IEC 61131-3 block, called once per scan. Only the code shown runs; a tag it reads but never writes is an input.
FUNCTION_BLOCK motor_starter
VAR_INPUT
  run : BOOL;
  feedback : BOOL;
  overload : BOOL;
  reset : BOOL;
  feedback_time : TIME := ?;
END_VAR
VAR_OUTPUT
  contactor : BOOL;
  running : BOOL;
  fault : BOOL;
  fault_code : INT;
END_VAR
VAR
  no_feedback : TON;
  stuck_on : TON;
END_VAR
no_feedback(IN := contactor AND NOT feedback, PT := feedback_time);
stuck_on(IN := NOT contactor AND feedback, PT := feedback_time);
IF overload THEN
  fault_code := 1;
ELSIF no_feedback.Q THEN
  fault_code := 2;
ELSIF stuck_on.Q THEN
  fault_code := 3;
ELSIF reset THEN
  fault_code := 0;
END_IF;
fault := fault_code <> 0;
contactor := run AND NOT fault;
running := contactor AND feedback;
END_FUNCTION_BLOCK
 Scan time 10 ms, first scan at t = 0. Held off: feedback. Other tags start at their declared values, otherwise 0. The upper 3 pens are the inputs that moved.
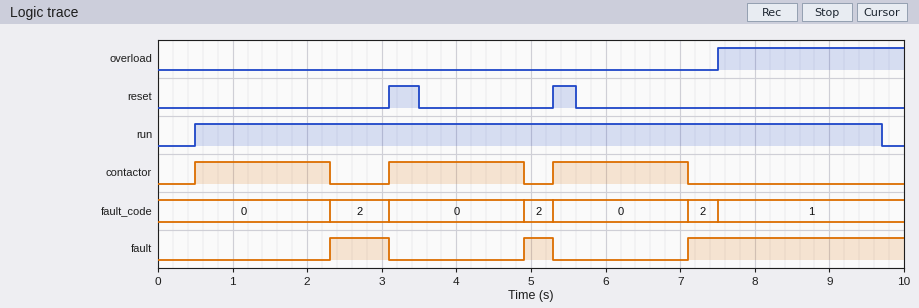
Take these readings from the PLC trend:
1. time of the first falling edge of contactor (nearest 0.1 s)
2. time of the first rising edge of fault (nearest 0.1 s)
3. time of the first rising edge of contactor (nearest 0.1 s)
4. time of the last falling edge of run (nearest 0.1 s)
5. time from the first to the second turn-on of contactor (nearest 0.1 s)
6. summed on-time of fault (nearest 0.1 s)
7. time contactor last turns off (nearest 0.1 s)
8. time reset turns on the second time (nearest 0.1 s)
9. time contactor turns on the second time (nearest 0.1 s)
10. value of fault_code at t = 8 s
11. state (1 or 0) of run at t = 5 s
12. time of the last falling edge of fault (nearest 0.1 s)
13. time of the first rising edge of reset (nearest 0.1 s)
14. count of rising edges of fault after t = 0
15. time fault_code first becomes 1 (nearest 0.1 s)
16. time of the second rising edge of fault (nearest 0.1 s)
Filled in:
2.3 s
2.3 s
0.5 s
9.7 s
2.6 s
4.1 s
7.1 s
5.3 s
3.1 s
1
1
5.3 s
3.1 s
3
7.5 s
4.9 s
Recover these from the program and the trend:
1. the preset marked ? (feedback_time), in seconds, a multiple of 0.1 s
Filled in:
1.8 s
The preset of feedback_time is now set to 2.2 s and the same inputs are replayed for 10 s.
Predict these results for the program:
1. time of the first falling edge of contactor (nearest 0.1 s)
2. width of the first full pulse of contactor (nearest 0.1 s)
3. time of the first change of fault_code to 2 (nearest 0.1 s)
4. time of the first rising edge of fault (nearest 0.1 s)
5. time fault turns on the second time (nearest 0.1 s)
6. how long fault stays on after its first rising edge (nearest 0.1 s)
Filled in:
2.7 s
2.2 s
2.7 s
2.7 s
5.3 s
0.4 s
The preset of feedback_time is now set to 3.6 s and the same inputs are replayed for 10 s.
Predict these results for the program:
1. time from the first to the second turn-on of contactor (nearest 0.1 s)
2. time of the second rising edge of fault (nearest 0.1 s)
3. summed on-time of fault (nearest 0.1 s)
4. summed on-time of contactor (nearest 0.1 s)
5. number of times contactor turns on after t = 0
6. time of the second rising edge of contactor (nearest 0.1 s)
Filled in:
4.8 s
7.5 s
3.7 s
5.8 s
2
5.3 s
